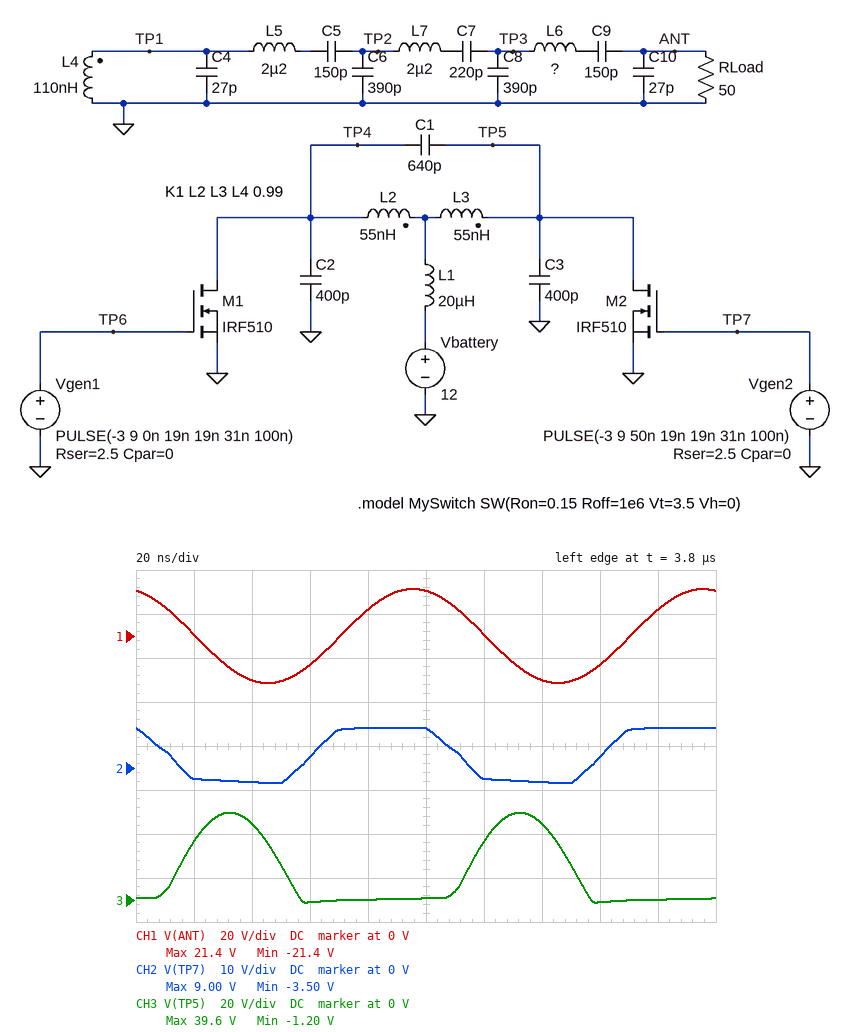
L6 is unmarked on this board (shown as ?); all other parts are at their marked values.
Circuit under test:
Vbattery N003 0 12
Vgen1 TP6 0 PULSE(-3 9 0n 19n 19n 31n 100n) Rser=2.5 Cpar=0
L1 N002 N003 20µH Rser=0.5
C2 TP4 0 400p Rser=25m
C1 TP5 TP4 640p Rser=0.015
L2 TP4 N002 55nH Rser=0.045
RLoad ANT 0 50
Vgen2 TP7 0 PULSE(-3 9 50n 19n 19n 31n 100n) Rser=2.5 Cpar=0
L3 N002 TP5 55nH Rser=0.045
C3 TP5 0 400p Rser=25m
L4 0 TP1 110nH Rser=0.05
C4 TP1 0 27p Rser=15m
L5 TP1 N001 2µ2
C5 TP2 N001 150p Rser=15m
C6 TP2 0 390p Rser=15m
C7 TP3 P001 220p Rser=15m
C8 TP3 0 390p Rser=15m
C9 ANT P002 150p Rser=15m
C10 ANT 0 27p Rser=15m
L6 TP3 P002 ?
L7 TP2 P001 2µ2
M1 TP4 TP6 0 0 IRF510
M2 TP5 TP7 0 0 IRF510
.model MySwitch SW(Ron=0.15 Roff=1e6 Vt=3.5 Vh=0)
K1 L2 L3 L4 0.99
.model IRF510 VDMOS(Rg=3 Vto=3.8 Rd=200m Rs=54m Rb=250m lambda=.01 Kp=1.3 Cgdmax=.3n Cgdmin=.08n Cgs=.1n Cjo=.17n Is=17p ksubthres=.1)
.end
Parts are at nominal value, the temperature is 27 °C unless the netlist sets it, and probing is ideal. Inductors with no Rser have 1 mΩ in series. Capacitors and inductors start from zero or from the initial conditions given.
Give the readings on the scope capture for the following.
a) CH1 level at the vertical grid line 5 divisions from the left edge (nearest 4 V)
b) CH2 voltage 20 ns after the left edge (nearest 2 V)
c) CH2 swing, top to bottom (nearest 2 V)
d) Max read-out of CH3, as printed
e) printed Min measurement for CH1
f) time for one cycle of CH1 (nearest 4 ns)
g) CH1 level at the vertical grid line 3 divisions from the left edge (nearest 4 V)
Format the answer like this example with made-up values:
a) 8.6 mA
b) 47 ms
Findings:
a) 20 V
b) -2 V
c) 12 V
d) 39.6 V
e) -21.4 V
f) 100 ns
g) -12 V
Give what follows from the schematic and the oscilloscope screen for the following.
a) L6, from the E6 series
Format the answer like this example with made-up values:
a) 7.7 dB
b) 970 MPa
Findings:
a) 3.3 µH
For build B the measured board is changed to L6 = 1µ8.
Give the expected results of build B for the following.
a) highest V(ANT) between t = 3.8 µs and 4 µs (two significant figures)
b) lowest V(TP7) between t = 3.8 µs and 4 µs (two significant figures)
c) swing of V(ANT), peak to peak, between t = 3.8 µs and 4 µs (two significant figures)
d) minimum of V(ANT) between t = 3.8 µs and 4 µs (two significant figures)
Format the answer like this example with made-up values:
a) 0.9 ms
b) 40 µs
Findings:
a) 20 V
b) -3.3 V
c) 40 V
d) -20 V
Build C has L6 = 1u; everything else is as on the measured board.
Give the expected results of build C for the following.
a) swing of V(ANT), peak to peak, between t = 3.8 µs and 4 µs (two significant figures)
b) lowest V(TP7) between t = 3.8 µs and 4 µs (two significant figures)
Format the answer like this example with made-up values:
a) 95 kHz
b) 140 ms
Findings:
a) 23 V
b) -3.3 V
